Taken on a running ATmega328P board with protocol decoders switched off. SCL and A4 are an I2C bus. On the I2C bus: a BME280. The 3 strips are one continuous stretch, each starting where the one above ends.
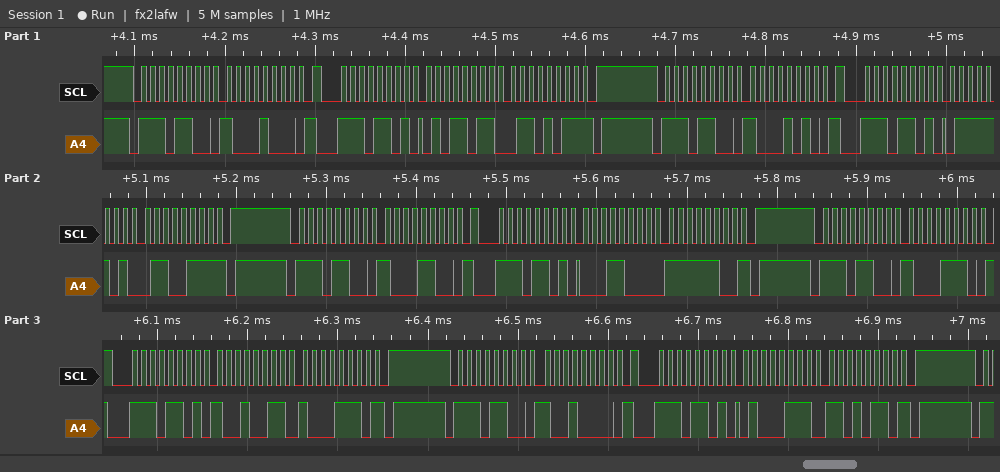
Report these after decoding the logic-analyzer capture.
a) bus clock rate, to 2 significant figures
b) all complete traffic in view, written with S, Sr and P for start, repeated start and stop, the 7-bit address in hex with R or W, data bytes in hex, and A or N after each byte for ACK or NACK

100 kHz
S 76W A 88 A Sr 76R A 5B A 6B N P S 76W A 8A A Sr 76R A 7D A 67 N P S 76W A 8C A Sr 76R A 18 A FC N P S 76W A 8E A Sr 76R A 93 A 8E N P S 76W A 90 A Sr 76R A 47 A D6 N P
